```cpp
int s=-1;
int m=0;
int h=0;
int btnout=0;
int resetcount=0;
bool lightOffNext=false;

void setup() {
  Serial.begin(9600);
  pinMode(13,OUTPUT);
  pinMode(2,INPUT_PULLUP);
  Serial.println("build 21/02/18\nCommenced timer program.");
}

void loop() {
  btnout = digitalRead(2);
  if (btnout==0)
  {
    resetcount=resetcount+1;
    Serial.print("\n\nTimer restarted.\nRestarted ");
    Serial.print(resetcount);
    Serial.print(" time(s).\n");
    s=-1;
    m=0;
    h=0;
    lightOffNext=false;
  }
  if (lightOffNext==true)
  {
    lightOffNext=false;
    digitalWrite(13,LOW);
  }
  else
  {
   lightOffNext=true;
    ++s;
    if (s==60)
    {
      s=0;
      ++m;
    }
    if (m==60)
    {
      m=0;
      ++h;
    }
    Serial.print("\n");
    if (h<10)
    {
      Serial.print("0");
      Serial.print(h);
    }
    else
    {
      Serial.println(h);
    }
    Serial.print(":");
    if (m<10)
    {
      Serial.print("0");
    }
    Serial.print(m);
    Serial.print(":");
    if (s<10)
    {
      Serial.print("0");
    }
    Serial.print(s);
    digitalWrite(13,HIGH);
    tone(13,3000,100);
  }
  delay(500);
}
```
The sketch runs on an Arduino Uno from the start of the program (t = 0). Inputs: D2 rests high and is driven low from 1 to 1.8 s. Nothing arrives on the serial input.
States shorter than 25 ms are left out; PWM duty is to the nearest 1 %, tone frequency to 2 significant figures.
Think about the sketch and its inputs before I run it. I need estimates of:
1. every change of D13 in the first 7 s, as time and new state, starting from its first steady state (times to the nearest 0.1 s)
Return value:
0 s tone 3000 Hz; 0.1 s low; 1 s tone 3000 Hz; 1.1 s low; 1.5 s tone 3000 Hz; 1.6 s low; 2.5 s tone 3000 Hz; 2.6 s low; 3.5 s tone 3000 Hz; 3.6 s low; 4.5 s tone 3000 Hz; 4.6 s low; 5.5 s tone 3000 Hz; 5.6 s low; 6.5 s tone 3000 Hz; 6.6 s low
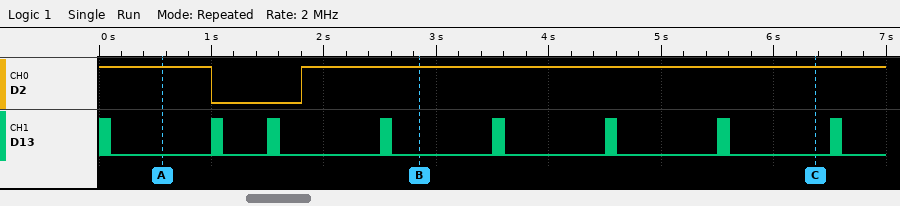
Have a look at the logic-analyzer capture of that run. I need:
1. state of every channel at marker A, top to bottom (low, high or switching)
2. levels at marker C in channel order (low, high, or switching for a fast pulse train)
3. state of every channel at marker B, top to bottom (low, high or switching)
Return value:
D2 high, D13 low
D2 high, D13 low
D2 high, D13 low
